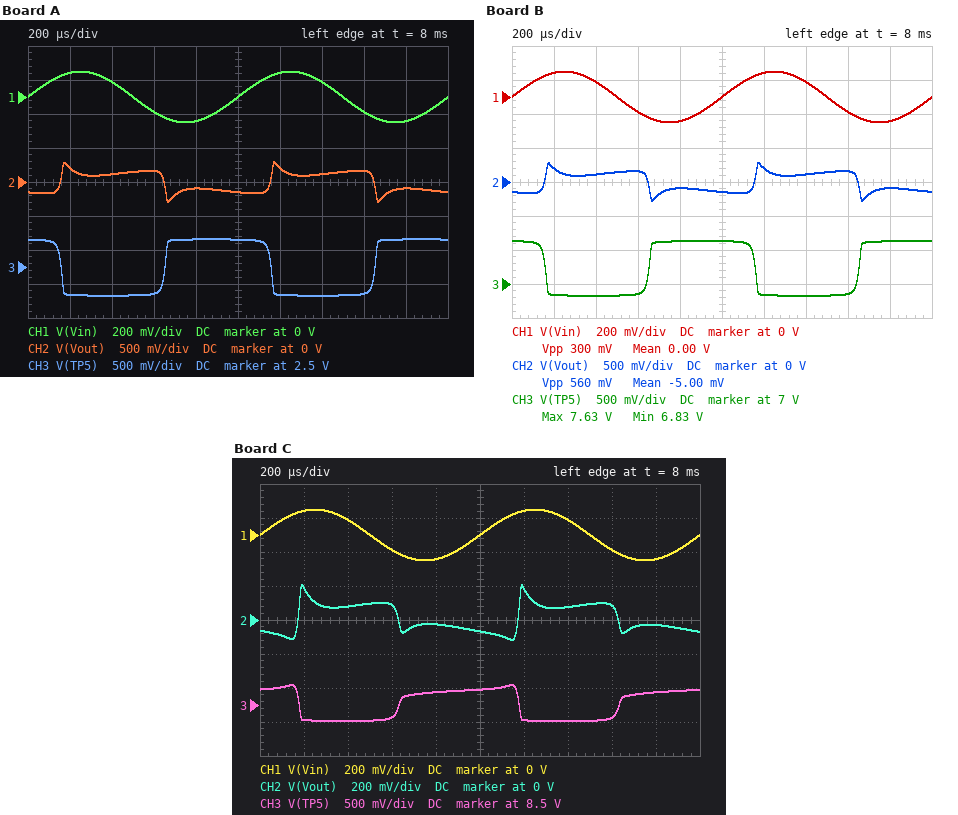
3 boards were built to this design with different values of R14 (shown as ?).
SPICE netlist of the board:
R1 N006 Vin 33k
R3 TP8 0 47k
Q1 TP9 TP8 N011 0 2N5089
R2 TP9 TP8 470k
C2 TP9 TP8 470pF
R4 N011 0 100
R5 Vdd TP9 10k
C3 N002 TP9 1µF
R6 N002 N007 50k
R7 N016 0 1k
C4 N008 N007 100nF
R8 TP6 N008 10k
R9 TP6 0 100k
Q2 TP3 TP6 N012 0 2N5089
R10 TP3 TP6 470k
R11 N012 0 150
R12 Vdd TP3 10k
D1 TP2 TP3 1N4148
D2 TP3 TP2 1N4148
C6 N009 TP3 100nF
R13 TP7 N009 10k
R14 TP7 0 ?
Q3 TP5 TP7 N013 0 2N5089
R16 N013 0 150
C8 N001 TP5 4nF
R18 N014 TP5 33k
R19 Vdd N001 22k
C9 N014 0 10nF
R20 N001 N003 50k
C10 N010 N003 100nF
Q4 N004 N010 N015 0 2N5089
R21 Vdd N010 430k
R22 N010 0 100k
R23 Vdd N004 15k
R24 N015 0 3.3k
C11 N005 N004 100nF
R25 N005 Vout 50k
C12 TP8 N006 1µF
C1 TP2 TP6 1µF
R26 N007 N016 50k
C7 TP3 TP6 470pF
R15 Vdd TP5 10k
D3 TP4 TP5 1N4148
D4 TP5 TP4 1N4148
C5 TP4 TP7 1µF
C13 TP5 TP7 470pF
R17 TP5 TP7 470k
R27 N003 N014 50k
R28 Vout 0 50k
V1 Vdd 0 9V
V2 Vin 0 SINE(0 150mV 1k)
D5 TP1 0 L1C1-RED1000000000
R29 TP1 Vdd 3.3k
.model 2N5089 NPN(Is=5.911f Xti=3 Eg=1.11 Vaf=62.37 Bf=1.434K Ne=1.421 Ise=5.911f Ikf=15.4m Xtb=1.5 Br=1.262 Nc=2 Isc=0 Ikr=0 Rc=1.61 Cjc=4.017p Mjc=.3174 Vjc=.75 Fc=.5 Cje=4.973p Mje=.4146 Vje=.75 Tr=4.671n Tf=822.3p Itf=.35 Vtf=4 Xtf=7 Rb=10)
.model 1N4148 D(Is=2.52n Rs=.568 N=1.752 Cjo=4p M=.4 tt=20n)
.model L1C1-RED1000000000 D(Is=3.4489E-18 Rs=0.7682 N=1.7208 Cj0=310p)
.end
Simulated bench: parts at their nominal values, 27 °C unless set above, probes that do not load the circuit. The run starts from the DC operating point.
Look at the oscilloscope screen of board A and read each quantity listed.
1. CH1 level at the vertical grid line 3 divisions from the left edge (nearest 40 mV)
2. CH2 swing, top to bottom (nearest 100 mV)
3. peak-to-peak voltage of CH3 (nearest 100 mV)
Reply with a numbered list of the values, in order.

1. -80 mV
2. 600 mV
3. 800 mV
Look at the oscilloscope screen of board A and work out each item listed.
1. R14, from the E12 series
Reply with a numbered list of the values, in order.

1. 270 kΩ
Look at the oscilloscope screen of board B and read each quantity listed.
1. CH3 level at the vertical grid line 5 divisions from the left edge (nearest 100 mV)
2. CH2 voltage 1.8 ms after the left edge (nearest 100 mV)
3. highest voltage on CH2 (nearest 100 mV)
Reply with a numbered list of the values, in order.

1. 7.6 V
2. -100 mV
3. 300 mV
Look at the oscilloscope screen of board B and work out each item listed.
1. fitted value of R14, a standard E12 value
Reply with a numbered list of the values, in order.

1. 47 kΩ
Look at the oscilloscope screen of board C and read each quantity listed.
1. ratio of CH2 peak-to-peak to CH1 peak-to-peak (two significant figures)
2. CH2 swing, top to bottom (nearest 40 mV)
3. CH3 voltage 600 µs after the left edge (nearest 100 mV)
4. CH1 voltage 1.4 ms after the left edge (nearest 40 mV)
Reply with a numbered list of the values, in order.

1. 1.1
2. 320 mV
3. 8.3 V
4. 80 mV
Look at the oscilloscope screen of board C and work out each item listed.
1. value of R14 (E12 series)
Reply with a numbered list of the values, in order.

1. 33 kΩ
